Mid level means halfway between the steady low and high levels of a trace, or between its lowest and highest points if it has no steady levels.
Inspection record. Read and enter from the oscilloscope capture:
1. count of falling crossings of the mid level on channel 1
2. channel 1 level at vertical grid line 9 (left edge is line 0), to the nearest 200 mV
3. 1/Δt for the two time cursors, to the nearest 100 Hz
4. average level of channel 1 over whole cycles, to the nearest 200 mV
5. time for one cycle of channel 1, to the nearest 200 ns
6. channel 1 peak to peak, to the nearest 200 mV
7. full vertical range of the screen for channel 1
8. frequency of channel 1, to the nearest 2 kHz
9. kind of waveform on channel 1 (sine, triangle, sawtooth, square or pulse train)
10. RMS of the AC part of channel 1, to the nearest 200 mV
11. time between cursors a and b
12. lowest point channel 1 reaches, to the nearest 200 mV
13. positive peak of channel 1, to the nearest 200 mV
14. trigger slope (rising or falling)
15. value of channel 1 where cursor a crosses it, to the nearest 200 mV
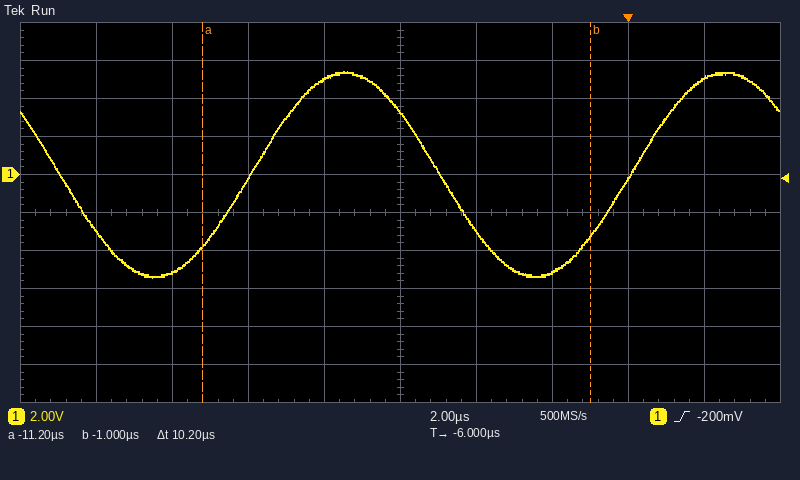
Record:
2
5.0 V
98.0 kHz
0.0 V
10.0 µs
10.8 V
20 V
100 kHz
sine
3.8 V
10.2 µs
-5.4 V
5.4 V
rising
-3.8 V
